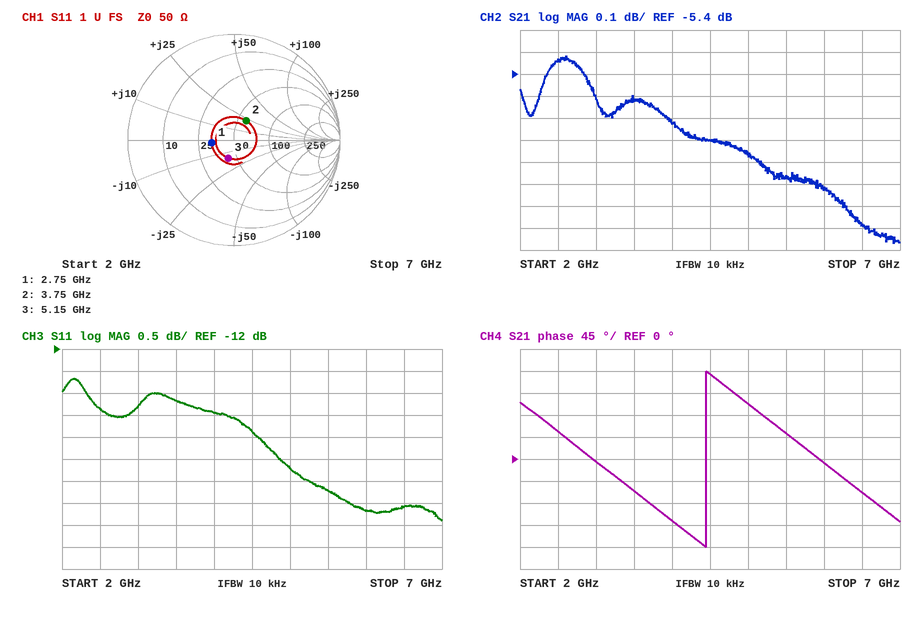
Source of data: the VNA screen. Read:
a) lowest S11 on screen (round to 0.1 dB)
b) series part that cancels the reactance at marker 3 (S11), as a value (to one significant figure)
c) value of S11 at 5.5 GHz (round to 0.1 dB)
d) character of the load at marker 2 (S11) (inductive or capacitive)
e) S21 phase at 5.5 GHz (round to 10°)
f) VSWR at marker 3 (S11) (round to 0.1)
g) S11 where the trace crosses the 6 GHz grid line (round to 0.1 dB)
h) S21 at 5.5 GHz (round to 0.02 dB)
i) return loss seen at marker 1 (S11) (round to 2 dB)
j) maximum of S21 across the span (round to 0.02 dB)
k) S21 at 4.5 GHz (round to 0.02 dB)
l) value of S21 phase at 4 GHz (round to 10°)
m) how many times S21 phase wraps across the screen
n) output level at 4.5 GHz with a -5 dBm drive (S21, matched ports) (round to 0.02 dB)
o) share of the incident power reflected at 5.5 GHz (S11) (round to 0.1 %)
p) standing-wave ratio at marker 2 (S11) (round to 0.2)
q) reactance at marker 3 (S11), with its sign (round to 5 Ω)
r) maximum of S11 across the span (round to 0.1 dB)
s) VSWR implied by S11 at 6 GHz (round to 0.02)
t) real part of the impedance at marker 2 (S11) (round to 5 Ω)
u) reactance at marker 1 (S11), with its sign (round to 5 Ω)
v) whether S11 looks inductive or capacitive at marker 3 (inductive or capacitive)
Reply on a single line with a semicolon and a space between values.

-15.9 dB; 500 pH; -15.2 dB; inductive; 50°; 1.4; -15.7 dB; -5.86 dB; 14 dB; -5.32 dB; -5.70 dB; -130°; 1; -10.70 dBm; 3.0 %; 1.6; -15 Ω; -12.7 dB; 1.40; 60 Ω; 0 Ω; capacitive
